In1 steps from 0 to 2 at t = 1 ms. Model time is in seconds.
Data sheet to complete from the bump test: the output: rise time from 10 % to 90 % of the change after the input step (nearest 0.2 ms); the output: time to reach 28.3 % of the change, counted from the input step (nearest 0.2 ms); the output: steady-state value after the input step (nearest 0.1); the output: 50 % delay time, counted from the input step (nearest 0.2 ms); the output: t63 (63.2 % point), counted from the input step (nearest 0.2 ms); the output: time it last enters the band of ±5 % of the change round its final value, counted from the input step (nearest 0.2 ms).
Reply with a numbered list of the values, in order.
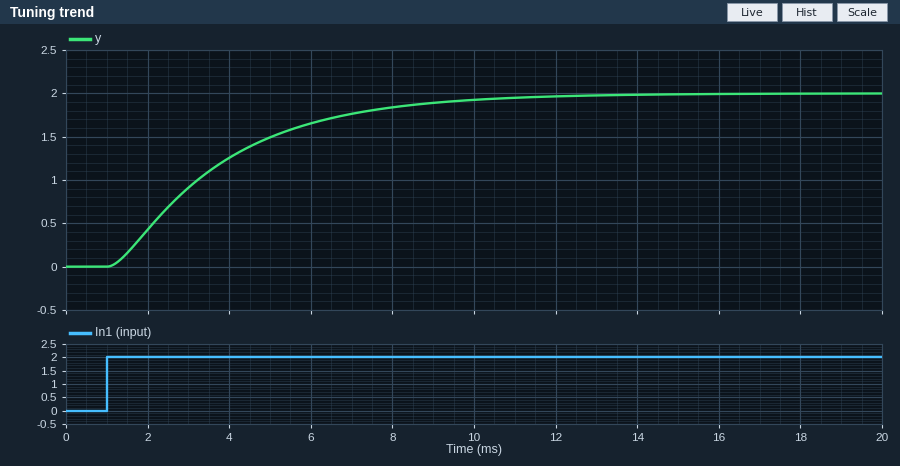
1. 5.8 ms
2. 1.2 ms
3. 2.0
4. 2.2 ms
5. 3.0 ms
6. 8.2 ms
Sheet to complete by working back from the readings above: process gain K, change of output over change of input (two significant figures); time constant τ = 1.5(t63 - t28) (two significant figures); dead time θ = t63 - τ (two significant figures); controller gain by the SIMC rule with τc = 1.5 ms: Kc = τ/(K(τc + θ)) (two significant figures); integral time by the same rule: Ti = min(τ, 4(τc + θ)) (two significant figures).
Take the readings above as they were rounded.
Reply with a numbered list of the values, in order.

1. 1.0
2. 2.7 ms
3. 0.30 ms
4. 1.5
5. 2.7 ms
